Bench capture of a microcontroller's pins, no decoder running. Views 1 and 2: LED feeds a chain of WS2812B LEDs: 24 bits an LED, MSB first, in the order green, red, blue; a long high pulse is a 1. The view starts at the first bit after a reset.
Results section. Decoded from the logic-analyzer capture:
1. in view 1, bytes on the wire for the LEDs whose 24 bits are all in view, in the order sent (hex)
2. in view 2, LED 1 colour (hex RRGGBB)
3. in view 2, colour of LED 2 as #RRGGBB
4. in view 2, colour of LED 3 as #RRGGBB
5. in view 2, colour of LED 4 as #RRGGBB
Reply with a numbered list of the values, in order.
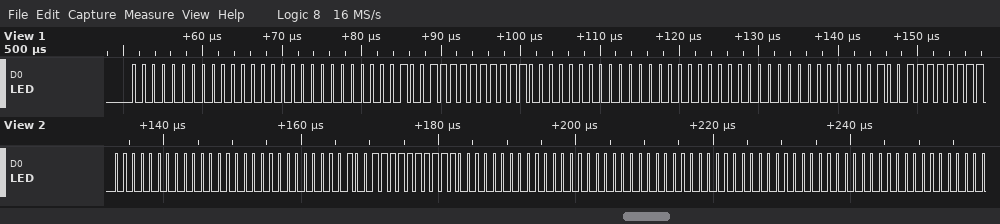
1. 00 00 00 13 FF 00 00 00 00
2. #000000
3. #FF1300
4. #000000
5. #000000
